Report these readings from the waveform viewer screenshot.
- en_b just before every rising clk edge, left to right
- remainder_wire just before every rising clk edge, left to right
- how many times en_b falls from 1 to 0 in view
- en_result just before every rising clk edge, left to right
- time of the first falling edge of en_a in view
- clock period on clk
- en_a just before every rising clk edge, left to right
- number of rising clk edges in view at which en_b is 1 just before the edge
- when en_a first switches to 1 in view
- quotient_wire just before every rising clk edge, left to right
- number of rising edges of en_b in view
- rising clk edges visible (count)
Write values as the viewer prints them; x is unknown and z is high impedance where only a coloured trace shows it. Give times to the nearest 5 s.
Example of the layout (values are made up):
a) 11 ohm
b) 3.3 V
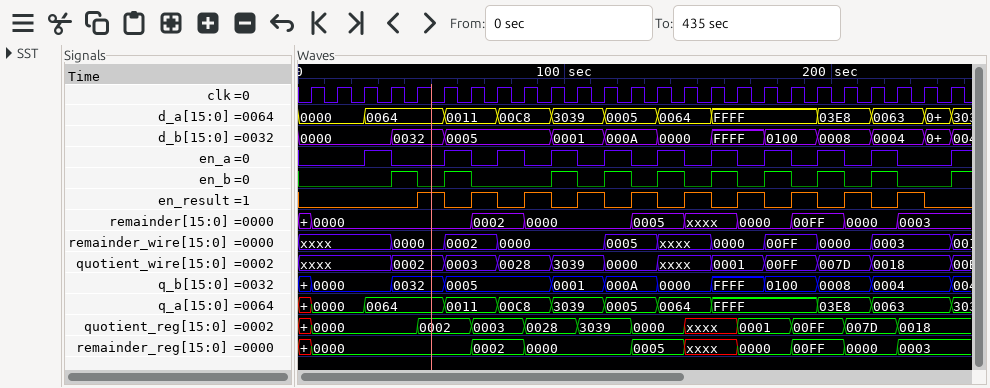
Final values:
a) 0 0 0 0 1 0 1 0 0 0 1 0 1 0 1 0 1 0 1 0 1 0 1 0 0
b) xxxx, xxxx, xxxx, xxxx, 0000, 0000, 0002, 0002, 0000, 0000, 0000, 0000, 0005, 0005, xxxx, xxxx, 0000, 0000, 00FF, 00FF, 0000, 0000, 0003, 0003, 0003
c) 9
d) 0 0 0 0 0 1 0 1 0 1 0 1 0 1 0 1 0 1 0 1 0 1 0 1 0
e) 35 s
f) 10 s
g) 0 0 0 1 0 0 1 0 1 0 1 0 1 0 1 0 1 0 1 0 1 0 1 0 0
h) 9
i) 25 s
j) xxxx, xxxx, xxxx, xxxx, 0002, 0002, 0003, 0003, 0028, 0028, 3039, 3039, 0000, 0000, xxxx, xxxx, 0001, 0001, 00FF, 00FF, 007D, 007D, 0018, 0018, 0018
k) 10
l) 25
